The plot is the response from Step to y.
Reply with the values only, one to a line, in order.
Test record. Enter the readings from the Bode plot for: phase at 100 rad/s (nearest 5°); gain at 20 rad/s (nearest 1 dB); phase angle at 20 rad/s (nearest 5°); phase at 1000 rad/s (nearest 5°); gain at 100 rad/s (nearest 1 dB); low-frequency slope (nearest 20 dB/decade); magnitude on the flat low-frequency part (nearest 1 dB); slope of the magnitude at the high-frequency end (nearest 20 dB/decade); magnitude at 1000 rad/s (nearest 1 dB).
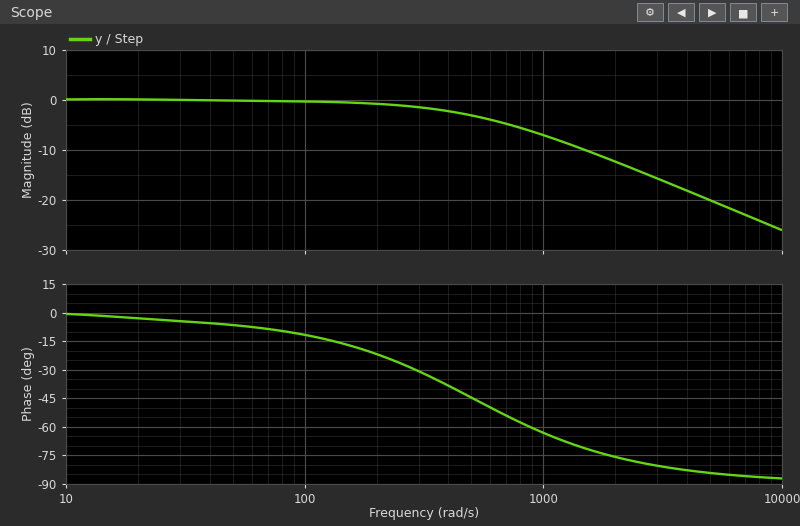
-10°
0 dB
-5°
-65°
0 dB
0 dB/decade
0 dB
-20 dB/decade
-7 dB
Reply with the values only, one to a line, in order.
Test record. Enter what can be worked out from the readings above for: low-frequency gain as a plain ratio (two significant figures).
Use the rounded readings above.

1.0
